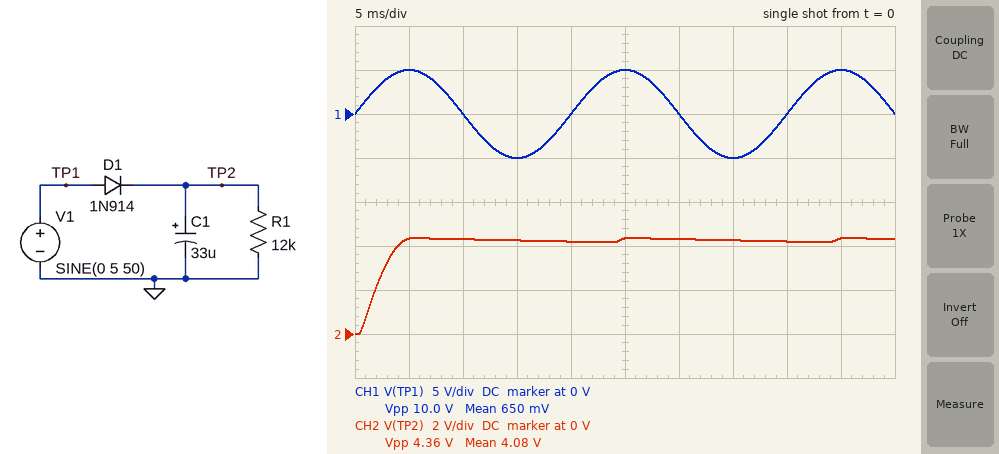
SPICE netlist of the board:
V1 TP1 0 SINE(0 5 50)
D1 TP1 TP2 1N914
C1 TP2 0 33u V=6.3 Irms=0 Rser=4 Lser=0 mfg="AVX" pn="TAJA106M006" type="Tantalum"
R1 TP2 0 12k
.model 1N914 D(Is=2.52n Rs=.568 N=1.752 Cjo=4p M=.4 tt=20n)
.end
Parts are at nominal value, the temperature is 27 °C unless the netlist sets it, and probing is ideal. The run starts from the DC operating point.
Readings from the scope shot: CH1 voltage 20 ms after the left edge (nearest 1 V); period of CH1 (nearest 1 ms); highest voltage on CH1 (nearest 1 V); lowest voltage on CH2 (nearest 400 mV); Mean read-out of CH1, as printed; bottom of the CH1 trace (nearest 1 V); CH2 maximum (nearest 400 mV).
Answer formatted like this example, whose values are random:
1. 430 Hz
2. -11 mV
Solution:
1. 0 V
2. 20 ms
3. 5 V
4. 0 V
5. 650 mV
6. -5 V
7. 4.4 V
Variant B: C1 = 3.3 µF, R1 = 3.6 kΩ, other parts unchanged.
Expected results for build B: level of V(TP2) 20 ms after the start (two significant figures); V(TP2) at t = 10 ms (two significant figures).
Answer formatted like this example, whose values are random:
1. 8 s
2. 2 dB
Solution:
1. 1.3 V
2. 3.0 V
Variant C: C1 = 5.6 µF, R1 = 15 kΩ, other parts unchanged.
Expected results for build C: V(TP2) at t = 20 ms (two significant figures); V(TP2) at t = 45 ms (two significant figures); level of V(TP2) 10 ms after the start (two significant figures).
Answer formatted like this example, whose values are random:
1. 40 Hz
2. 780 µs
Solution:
1. 3.7 V
2. 4.4 V
3. 4.2 V
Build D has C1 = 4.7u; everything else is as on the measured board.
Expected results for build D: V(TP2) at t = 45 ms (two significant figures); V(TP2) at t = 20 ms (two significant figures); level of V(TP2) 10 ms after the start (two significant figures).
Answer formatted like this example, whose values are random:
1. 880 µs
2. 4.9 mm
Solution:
1. 4.4 V
2. 3.4 V
3. 4.1 V
